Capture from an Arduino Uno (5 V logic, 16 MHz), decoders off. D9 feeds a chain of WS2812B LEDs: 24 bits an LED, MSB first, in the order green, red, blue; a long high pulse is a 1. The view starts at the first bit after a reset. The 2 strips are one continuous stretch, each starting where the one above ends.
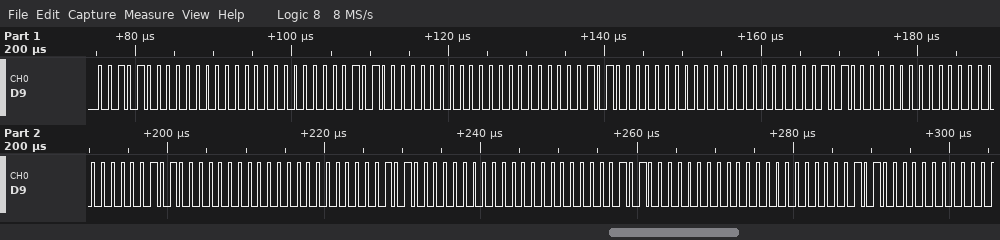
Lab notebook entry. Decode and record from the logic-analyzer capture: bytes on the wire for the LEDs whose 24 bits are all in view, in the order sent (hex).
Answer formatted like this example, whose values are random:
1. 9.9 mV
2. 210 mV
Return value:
1. 28 00 00 28 00 00 28 00 00 28 00 00 28 00 00 28 00 00 28 00 00
